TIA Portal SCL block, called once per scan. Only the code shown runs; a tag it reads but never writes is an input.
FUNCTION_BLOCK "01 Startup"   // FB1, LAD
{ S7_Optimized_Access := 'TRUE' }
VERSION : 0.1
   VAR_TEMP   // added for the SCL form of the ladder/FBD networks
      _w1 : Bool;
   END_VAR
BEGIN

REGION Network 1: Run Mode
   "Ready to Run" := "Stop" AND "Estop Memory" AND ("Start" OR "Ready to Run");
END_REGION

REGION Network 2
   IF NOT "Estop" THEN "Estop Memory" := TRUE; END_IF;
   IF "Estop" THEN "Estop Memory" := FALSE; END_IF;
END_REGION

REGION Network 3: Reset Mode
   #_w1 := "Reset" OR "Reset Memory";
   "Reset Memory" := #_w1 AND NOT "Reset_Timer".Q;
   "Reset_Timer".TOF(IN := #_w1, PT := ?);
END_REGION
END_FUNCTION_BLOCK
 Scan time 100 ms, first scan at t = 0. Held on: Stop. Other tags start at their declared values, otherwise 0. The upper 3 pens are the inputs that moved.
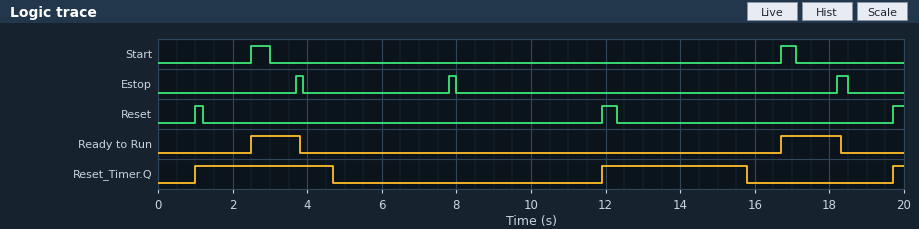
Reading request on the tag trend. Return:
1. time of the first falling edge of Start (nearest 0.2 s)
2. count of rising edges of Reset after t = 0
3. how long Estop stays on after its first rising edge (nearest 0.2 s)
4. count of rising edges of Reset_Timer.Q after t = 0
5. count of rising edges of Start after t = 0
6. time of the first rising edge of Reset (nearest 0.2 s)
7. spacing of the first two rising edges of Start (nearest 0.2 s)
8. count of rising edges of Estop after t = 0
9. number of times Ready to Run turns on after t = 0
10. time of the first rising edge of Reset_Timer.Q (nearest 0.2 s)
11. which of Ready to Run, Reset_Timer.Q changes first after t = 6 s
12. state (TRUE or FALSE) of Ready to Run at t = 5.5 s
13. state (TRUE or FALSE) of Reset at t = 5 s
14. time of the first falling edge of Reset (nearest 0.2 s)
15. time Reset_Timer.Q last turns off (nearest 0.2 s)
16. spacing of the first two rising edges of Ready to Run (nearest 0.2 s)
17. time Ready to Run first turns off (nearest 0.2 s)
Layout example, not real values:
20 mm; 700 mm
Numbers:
3.0 s; 3; 0.2 s; 3; 2; 1.0 s; 14.2 s; 3; 2; 1.0 s; Reset_Timer.Q; FALSE; FALSE; 1.2 s; 15.8 s; 14.2 s; 3.8 s
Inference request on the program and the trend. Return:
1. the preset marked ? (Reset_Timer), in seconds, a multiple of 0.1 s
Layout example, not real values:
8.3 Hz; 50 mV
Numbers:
3.5 s
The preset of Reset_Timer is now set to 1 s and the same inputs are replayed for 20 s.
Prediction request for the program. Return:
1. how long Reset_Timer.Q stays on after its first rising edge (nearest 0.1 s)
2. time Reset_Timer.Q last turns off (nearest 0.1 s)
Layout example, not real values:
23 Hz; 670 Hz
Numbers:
1.2 s; 13.3 s
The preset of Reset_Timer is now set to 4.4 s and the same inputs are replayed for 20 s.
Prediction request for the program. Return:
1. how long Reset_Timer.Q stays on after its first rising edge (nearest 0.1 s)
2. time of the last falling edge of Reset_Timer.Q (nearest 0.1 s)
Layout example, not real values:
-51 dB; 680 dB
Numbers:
4.6 s; 16.7 s
